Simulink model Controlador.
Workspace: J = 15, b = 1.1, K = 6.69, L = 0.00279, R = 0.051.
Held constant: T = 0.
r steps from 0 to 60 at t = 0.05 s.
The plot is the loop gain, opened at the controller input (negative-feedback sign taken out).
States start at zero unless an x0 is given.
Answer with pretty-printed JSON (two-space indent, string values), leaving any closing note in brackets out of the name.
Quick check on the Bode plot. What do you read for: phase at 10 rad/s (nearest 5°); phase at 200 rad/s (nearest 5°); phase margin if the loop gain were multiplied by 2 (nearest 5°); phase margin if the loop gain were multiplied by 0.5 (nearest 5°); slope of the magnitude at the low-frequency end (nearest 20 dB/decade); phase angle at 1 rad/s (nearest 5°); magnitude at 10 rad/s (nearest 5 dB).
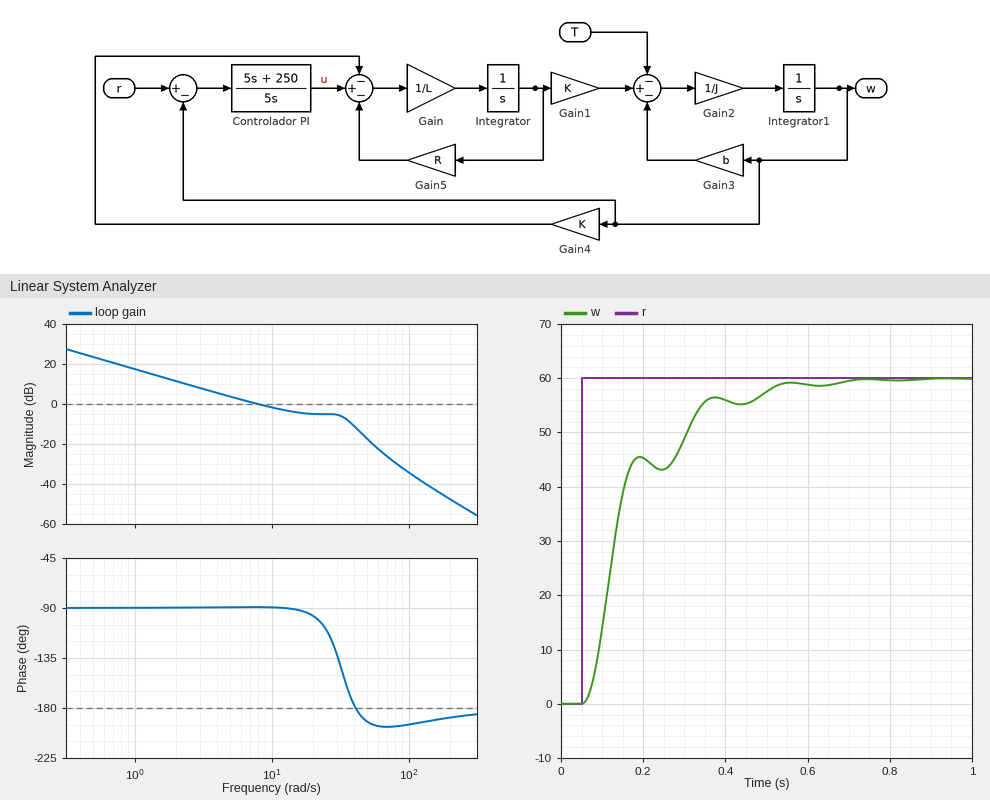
{
  "phase at 10 rad/s": "-90°",
  "phase at 200 rad/s": "-190°",
  "phase margin if the loop gain were multiplied by 2": "35°",
  "phase margin if the loop gain were multiplied by 0.5": "90°",
  "slope of the magnitude at the low-frequency end": "-20 dB/decade",
  "phase angle at 1 rad/s": "-90°",
  "magnitude at 10 rad/s": "0 dB"
}
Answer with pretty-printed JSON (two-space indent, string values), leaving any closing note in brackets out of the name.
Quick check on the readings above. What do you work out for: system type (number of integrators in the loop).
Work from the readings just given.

{
  "system type": "1"
}
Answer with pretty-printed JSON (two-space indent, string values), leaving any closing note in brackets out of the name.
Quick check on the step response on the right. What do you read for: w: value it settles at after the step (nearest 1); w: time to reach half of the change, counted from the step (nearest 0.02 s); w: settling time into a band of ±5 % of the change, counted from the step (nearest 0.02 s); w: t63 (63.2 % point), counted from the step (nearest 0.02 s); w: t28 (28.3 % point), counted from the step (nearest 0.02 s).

{
  "w: value it settles at after the step": "60",
  "w: time to reach half of the change, counted from the step": "0.08 s",
  "w: settling time into a band of ±5 % of the change, counted from the step": "0.44 s",
  "w: t63 (63.2 % point), counted from the step": "0.10 s",
  "w: t28 (28.3 % point), counted from the step": "0.06 s"
}
